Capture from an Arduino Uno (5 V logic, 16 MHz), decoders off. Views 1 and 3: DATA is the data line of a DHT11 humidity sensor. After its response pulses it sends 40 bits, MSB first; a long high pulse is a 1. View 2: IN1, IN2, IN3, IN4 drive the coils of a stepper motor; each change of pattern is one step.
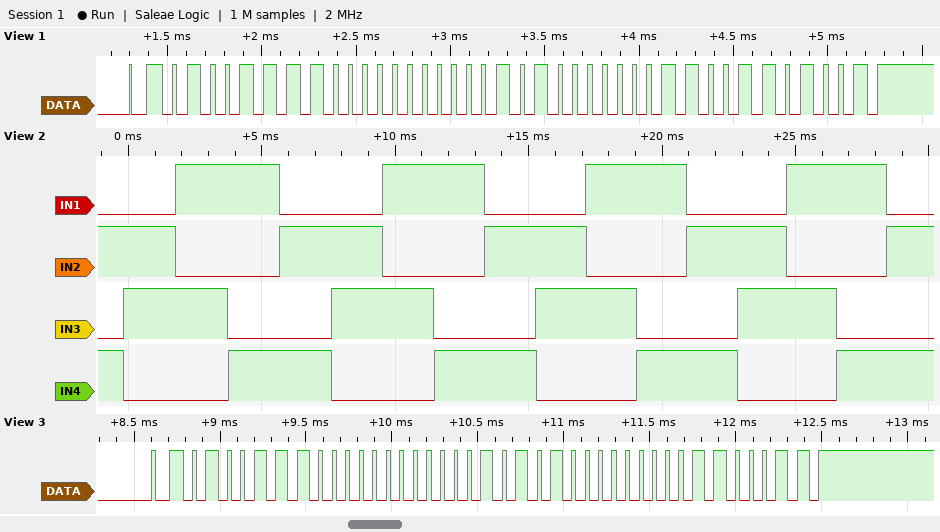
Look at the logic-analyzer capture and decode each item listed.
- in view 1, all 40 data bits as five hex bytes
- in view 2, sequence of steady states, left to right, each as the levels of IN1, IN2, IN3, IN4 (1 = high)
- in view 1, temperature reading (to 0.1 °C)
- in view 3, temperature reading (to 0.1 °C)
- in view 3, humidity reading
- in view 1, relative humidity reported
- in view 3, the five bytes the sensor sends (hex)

4F 00 14 06 69
0101 0110 1010 1001 0101 0110 1010 1001 0101 0110 1010 1001 0101 0110 1010 1001 0101
20.6 °C
21.0 °C
78 %
79 %
4E 00 15 00 63
